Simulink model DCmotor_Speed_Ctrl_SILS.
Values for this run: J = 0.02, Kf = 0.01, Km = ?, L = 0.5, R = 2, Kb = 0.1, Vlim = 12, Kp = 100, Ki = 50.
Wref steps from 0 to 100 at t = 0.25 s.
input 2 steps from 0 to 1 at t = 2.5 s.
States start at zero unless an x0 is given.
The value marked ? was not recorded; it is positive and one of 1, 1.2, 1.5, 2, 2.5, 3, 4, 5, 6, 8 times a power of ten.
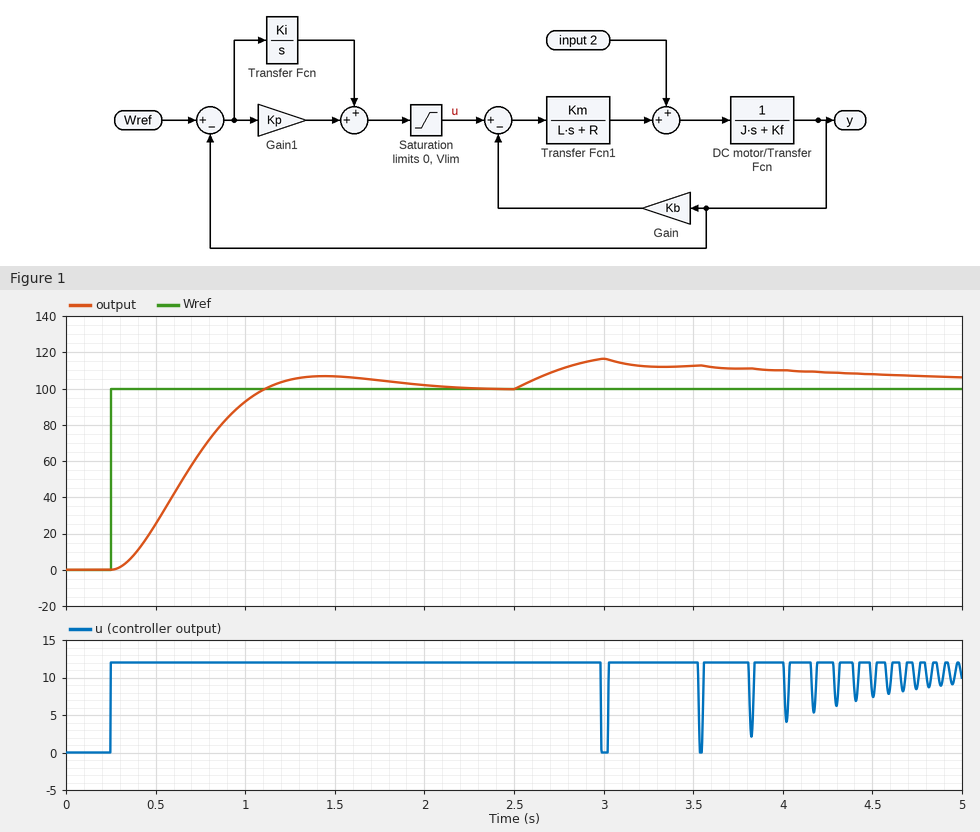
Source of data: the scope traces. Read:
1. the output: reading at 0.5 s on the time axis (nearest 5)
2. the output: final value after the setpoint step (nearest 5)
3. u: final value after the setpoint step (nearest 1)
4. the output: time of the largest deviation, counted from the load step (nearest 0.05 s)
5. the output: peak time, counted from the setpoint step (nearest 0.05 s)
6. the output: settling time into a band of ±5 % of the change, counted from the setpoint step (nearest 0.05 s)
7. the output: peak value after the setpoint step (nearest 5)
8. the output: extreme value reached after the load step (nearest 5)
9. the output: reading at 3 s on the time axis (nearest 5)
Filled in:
25
100
12
0.50 s
1.20 s
1.45 s
105
115
115
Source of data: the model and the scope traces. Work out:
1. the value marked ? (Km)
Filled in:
1
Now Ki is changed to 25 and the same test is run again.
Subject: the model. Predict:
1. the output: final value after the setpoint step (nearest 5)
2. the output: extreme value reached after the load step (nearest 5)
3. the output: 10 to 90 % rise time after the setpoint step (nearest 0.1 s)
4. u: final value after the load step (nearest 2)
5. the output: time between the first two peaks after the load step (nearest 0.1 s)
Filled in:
100
110
0.6 s
10
0.5 s
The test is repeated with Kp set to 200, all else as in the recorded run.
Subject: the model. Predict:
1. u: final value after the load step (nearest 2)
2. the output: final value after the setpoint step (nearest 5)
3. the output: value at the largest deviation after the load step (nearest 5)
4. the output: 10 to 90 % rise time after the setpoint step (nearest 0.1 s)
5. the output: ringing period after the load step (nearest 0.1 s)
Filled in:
10
100
110
0.6 s
0.5 s
